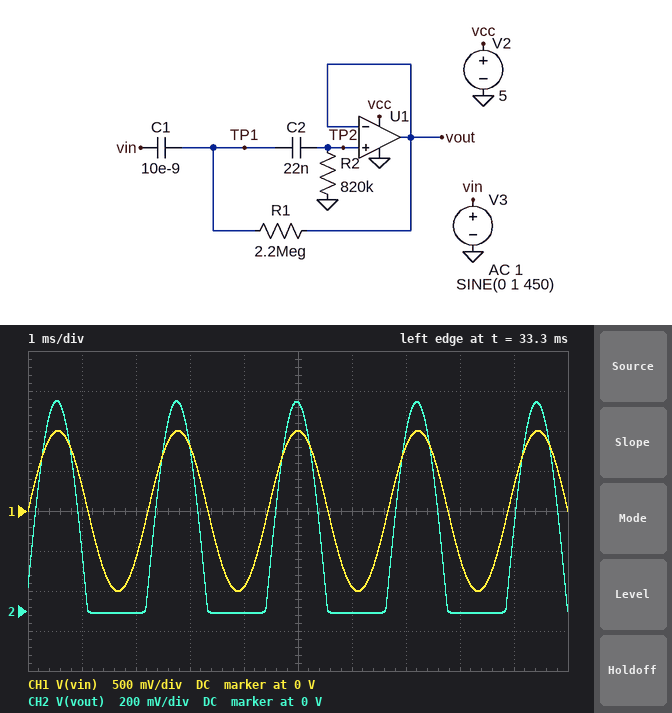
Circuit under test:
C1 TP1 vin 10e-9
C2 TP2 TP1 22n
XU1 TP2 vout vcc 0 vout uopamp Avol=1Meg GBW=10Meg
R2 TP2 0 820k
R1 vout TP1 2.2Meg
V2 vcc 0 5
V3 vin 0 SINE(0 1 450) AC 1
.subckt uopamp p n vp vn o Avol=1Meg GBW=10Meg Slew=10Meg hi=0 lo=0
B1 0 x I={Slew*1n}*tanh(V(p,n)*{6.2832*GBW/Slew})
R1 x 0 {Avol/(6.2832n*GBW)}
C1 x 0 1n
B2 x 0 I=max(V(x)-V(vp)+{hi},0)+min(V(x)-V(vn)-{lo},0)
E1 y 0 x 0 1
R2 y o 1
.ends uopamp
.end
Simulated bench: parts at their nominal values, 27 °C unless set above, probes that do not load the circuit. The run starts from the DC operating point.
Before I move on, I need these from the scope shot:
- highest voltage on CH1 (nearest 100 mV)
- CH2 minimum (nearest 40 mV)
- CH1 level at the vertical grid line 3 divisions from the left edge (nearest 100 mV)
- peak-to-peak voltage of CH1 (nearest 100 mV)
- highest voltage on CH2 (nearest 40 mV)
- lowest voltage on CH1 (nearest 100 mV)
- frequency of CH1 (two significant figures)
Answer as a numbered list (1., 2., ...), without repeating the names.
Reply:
1. 1.0 V
2. 0 V
3. 800 mV
4. 2.0 V
5. 1.04 V
6. -1.0 V
7. 450 Hz
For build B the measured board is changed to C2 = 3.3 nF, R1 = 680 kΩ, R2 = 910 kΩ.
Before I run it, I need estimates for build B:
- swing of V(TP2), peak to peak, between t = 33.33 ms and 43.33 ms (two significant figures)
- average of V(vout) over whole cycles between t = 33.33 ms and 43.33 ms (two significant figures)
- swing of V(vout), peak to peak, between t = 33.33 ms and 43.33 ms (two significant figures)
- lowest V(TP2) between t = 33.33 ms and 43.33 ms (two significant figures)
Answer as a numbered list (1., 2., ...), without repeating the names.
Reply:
1. 2.0 V
2. 310 mV
3. 1.0 V
4. -990 mV
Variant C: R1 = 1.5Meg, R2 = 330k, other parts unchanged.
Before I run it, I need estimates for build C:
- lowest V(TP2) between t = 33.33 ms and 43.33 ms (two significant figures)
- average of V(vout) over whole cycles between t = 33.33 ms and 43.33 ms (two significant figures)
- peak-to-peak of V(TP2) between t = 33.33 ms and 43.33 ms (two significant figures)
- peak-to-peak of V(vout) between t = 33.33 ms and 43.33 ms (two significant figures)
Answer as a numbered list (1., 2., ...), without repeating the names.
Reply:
1. -970 mV
2. 320 mV
3. 2.0 V
4. 1.0 V
